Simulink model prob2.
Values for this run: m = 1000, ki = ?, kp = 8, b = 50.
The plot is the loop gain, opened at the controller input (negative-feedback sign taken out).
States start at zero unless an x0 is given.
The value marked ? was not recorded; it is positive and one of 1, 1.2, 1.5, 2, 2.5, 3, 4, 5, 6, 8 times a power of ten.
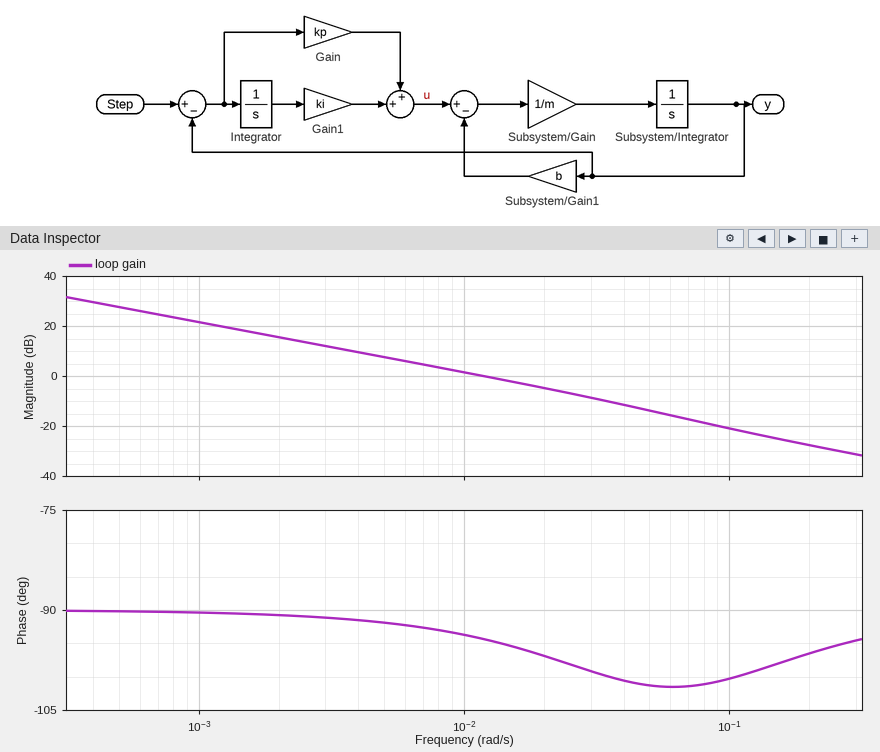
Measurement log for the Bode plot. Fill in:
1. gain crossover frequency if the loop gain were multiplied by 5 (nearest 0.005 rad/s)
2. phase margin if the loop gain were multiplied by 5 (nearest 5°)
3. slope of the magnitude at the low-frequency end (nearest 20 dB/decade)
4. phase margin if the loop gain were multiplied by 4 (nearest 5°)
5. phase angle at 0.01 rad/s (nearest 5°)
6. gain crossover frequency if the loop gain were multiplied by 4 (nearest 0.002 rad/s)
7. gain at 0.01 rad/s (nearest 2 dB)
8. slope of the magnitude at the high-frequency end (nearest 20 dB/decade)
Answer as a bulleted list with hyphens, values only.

- 0.050 rad/s
- 80°
- -20 dB/decade
- 80°
- -95°
- 0.042 rad/s
- 2 dB
- -20 dB/decade
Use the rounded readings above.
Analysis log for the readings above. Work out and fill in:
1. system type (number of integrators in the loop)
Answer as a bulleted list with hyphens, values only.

- 1
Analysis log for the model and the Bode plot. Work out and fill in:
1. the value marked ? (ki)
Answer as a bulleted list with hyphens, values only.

- 0.6
